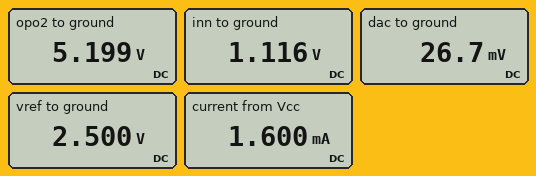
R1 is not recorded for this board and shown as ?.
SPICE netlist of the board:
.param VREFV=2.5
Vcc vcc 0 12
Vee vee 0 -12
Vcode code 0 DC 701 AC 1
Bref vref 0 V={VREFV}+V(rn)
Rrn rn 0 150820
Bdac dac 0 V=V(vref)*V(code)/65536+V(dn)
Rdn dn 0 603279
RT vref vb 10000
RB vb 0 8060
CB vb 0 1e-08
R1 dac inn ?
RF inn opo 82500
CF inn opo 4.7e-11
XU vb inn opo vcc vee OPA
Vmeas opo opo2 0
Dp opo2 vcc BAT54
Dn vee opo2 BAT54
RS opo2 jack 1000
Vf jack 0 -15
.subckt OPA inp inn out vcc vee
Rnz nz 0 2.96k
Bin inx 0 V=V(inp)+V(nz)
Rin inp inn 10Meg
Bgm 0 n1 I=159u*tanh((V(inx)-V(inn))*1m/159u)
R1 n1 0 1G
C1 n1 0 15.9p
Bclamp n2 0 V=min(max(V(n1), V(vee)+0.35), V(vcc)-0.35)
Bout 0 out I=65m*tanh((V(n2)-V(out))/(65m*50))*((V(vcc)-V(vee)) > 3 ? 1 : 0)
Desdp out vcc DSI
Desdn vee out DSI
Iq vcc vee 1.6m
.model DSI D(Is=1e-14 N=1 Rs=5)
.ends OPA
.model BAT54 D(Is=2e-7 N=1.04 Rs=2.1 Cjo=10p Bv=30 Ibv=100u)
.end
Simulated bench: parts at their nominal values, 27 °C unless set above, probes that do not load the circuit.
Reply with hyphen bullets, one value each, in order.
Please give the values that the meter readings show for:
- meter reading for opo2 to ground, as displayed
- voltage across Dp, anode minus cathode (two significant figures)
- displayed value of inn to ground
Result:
- 5.199 V
- -6.8 V
- 1.116 V
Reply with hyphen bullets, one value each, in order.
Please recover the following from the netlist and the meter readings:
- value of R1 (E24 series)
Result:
- 22 kΩ
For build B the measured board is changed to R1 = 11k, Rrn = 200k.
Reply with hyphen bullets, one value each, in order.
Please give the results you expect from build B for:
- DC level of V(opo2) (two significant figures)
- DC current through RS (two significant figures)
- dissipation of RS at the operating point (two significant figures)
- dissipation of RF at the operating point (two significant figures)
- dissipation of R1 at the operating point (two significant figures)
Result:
- 9.3 V
- 24 mA
- 590 mW
- 810 µW
- 110 µW
